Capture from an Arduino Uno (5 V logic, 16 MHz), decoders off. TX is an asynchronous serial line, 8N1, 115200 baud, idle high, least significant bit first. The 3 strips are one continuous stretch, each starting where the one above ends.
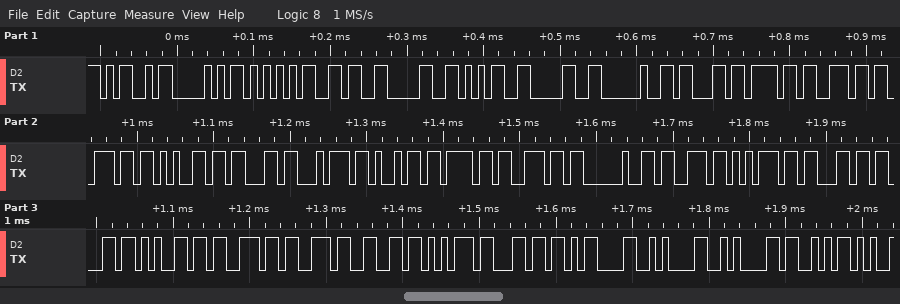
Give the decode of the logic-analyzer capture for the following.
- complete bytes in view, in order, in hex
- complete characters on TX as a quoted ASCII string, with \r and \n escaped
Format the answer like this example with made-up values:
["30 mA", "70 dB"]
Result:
["4D 50 55 36 30 35 30 20 63 6F 6E 6E 65 63 74 69 6F 6E 20 73 75 63 63 65 73 73 66 75 6C 0D 0A 0A 53", "\"MPU6050 connection successful\\r\\n\\nS\""]
